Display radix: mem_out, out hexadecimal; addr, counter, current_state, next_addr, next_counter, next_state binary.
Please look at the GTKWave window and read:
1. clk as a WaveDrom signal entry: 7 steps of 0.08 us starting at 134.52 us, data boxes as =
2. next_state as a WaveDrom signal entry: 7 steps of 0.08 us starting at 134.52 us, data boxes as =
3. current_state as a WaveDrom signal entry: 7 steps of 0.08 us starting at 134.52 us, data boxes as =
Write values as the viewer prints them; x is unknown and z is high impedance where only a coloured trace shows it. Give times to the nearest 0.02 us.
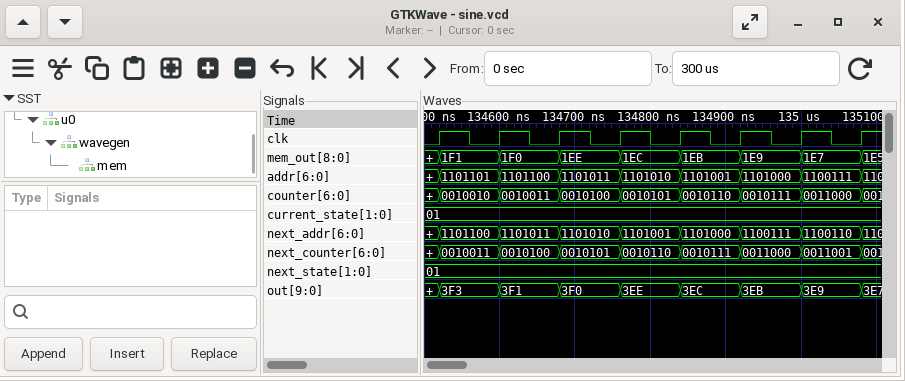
{name: 'clk', wave: 'p......'}
{name: 'next_state', wave: '=......', data: '01'}
{name: 'current_state', wave: '=......', data: '01'}
